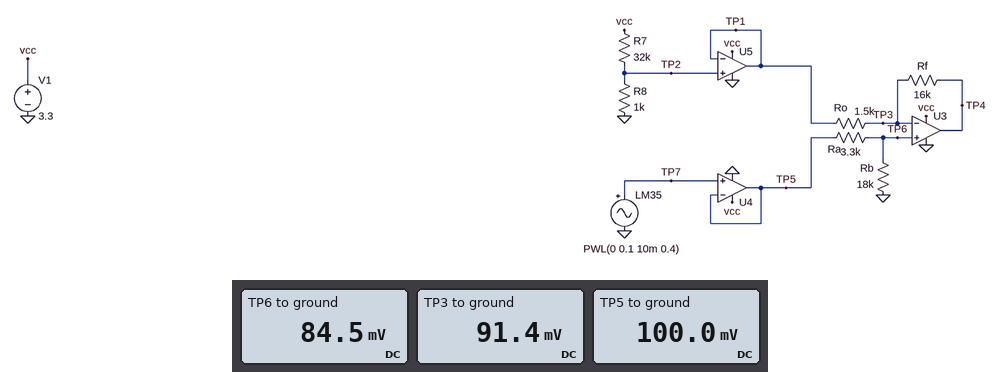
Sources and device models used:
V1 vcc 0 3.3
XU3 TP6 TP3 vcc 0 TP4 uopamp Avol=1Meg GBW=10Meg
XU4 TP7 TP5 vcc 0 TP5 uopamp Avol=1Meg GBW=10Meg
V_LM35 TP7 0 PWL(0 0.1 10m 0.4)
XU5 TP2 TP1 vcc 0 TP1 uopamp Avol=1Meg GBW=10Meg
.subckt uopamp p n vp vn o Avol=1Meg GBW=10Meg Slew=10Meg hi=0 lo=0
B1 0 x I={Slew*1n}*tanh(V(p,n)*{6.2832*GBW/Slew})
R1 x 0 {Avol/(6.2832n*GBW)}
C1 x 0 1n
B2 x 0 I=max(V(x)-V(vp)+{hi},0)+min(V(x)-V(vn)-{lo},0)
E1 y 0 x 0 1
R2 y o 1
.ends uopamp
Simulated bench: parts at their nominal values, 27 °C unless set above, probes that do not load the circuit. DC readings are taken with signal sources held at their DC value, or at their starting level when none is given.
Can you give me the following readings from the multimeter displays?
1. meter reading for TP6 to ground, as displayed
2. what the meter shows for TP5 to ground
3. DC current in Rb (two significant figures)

84.5 mV
100.0 mV
4.7 µA
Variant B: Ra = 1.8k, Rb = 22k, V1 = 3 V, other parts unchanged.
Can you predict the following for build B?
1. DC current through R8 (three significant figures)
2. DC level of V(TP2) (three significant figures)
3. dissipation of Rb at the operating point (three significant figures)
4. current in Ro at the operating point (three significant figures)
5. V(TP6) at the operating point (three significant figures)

90.9 µA
90.9 mV
388 nW
1.02 µA
92.4 mV
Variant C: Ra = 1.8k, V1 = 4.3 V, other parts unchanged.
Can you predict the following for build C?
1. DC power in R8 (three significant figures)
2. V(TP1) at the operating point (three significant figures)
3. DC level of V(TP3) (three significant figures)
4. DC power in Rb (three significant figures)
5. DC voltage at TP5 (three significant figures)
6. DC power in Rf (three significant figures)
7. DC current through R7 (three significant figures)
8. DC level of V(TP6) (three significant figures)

17.0 µW
130 mV
119 mV
459 nW
100 mV
911 nW
130 µA
90.9 mV
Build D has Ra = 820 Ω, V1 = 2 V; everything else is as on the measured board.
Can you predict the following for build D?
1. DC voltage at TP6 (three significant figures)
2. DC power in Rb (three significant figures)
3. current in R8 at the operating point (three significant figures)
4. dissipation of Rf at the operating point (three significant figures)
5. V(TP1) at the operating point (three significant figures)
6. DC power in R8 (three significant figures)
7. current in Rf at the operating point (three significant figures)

95.6 mV
508 nW
60.6 µA
8.73 µW
60.6 mV
3.67 µW
23.4 µA
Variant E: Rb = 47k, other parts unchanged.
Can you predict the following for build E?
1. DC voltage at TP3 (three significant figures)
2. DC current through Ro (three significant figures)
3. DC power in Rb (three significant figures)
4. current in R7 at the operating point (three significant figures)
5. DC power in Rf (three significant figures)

93.4 mV
4.37 µA
186 nW
100 µA
306 nW
